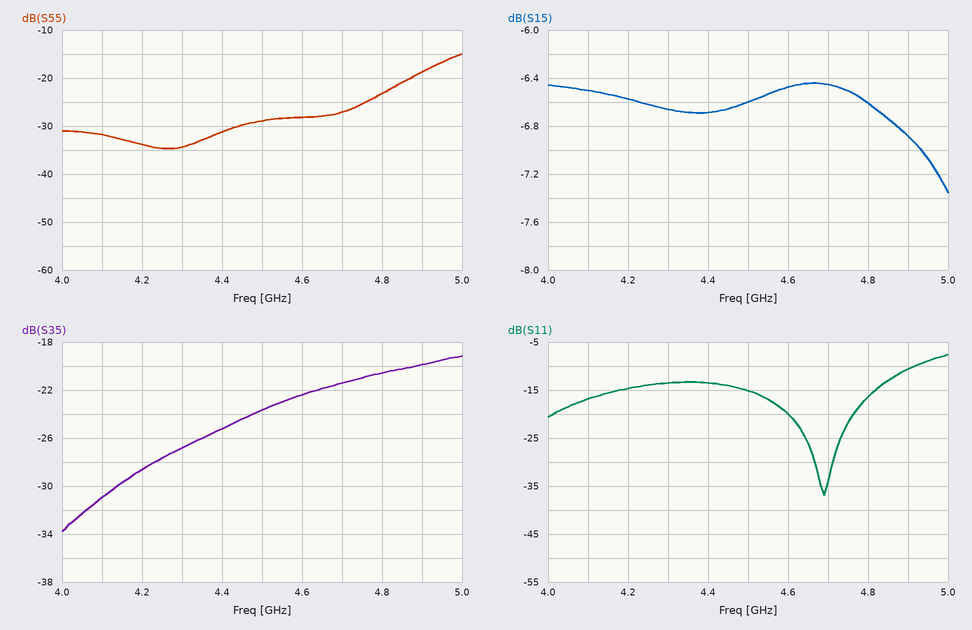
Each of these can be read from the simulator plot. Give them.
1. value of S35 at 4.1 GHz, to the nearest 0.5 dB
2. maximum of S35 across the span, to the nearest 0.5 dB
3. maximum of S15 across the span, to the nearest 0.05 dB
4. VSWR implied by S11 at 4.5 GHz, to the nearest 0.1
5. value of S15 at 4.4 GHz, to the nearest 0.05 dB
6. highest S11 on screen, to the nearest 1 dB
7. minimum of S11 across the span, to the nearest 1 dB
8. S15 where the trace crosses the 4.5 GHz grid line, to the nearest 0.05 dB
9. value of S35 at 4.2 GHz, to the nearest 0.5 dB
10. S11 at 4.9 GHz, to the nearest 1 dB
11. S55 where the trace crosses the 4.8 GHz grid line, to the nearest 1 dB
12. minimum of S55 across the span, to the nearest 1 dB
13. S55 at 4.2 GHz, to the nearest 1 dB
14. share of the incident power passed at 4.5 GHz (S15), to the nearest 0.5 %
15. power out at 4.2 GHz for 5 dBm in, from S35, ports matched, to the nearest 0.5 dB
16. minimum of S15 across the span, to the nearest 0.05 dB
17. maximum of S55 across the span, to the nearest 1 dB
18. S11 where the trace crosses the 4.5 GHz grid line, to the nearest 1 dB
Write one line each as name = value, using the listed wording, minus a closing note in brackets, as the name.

value of S35 at 4.1 GHz, to the nearest 0.5 dB = -31.0 dB
maximum of S35 across the span, to the nearest 0.5 dB = -19.0 dB
maximum of S15 across the span, to the nearest 0.05 dB = -6.45 dB
VSWR implied by S11 at 4.5 GHz, to the nearest 0.1 = 1.4
value of S15 at 4.4 GHz, to the nearest 0.05 dB = -6.70 dB
highest S11 on screen, to the nearest 1 dB = -8 dB
minimum of S11 across the span, to the nearest 1 dB = -37 dB
S15 where the trace crosses the 4.5 GHz grid line, to the nearest 0.05 dB = -6.60 dB
value of S35 at 4.2 GHz, to the nearest 0.5 dB = -28.5 dB
S11 at 4.9 GHz, to the nearest 1 dB = -11 dB
S55 where the trace crosses the 4.8 GHz grid line, to the nearest 1 dB = -23 dB
minimum of S55 across the span, to the nearest 1 dB = -35 dB
S55 at 4.2 GHz, to the nearest 1 dB = -34 dB
share of the incident power passed at 4.5 GHz (S15), to the nearest 0.5 % = 22.0 %
power out at 4.2 GHz for 5 dBm in, from S35, ports matched, to the nearest 0.5 dB = -23.5 dBm
minimum of S15 across the span, to the nearest 0.05 dB = -7.35 dB
maximum of S55 across the span, to the nearest 1 dB = -15 dB
S11 where the trace crosses the 4.5 GHz grid line, to the nearest 1 dB = -15 dB
